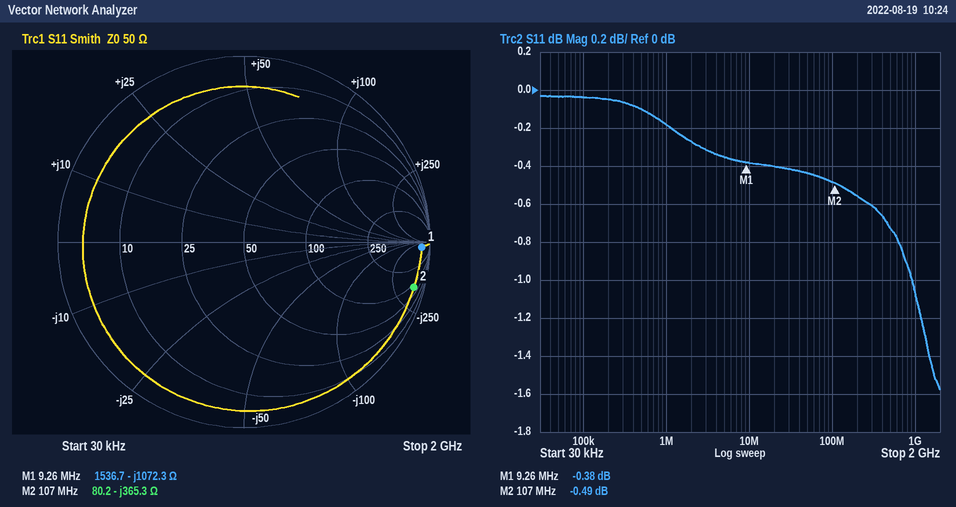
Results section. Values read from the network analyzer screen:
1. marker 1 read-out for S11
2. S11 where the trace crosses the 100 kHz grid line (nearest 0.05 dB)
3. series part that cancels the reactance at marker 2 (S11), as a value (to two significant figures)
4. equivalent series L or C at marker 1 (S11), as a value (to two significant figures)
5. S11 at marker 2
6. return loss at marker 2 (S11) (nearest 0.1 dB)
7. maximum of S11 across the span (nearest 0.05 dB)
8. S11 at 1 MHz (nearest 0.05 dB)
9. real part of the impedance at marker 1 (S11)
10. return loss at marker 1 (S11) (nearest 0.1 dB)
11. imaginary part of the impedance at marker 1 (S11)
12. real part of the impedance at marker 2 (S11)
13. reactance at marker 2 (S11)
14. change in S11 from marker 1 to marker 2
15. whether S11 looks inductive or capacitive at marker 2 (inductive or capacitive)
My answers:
-0.38 dB
-0.05 dB
540 nH
16 pF
-0.49 dB
0.5 dB
-0.05 dB
-0.20 dB
1536.7 Ω
0.4 dB
-1072.3 Ω
80.2 Ω
-365.3 Ω
-0.11 dB
capacitive
